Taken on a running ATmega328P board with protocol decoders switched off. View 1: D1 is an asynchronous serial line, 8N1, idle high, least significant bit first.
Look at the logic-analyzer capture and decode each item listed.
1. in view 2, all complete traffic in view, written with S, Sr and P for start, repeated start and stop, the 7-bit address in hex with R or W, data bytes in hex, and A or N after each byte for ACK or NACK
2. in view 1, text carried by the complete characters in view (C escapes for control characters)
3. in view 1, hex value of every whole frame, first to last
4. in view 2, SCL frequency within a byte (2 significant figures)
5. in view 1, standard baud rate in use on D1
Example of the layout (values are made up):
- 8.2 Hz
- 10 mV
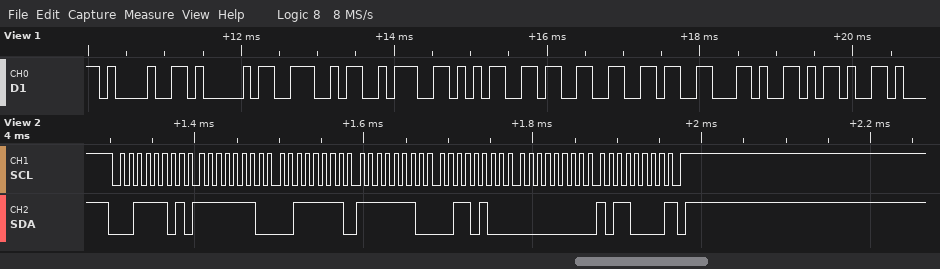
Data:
- S 1ER A FE A 3F A FE A 34 A 00 A B0 N P
- "!AN:536,-"
- 21 41 4E 3A 35 33 36 2C 2D
- 100 kHz
- 9600 baud
